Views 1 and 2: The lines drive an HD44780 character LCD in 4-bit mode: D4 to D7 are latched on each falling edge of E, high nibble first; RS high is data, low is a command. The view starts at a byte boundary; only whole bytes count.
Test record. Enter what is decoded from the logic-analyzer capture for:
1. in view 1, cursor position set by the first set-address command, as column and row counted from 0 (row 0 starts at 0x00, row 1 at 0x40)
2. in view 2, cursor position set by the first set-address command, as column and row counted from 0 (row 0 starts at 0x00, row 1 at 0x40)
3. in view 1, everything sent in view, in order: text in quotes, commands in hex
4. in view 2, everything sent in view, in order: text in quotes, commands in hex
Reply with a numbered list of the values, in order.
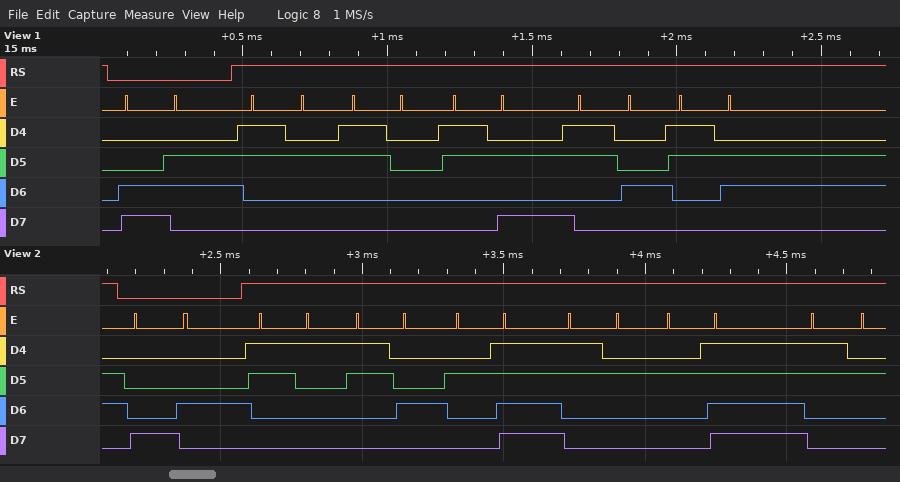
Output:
1. column 6, row 1
2. column 4, row 0
3. 0xC6 "20:46"
4. 0x84 "14/2/2"
